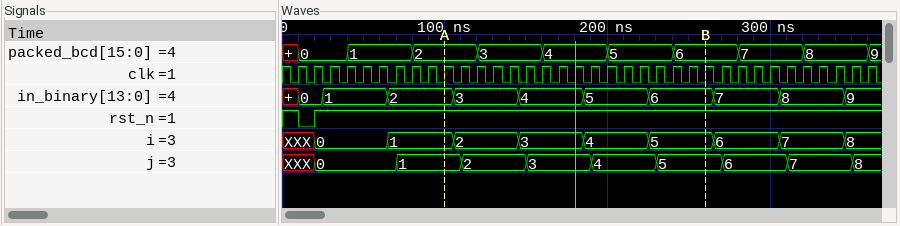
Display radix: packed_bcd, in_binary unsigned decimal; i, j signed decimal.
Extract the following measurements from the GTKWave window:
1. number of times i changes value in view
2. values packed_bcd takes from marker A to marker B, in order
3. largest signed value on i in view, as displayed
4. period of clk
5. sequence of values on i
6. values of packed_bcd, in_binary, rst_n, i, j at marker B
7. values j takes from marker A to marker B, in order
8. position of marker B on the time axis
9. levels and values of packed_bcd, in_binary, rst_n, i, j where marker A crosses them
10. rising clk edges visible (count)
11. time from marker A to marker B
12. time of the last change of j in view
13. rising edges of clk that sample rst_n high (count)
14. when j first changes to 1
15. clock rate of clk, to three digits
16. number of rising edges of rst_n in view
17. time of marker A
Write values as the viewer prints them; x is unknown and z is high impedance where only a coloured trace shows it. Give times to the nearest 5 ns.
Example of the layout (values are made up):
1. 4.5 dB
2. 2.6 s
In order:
1. 9
2. 2, 3, 4, 5, 6
3. 8
4. 10 ns
5. XXX, 0, 1, 2, 3, 4, 5, 6, 7, 8
6. packed_bcd=6, in_binary=6, rst_n=1, i=5, j=5
7. 1, 2, 3, 4, 5
8. 260 ns
9. packed_bcd=2, in_binary=2, rst_n=1, i=1, j=1
10. 36
11. 160 ns
12. 350 ns
13. 35
14. 70 ns
15. 100 MHz
16. 1
17. 100 ns
